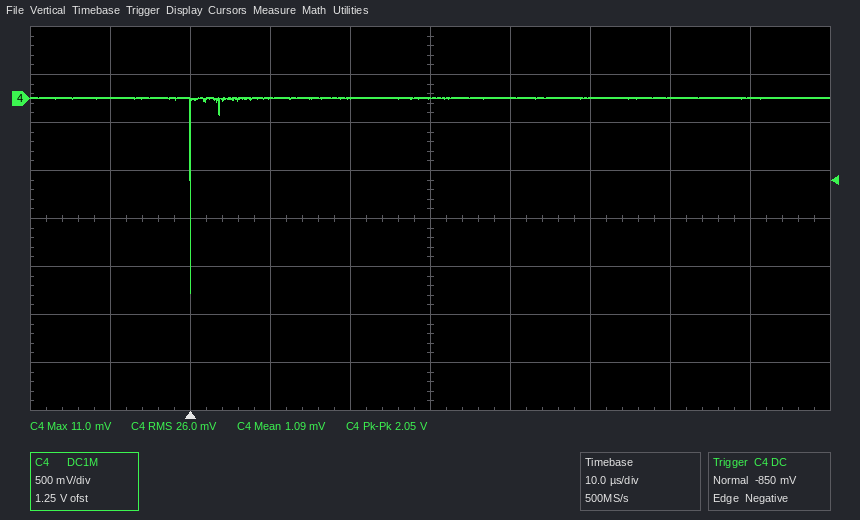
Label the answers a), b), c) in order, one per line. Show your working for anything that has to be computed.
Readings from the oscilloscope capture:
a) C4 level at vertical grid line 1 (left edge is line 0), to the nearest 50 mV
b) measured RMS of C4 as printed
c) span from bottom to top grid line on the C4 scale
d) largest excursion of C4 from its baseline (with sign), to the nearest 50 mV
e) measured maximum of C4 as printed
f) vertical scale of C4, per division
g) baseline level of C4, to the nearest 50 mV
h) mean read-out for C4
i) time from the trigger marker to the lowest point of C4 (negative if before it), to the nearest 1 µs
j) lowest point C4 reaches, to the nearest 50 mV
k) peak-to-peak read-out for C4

a) 0 mV
b) 26.0 mV
c) 4 V
d) -2.05 V − (0 mV) = -2.05 V
e) 11.0 mV
f) 500 mV
g) 0 mV
h) 1.09 mV
i) 0 µs
j) -2.05 V
k) 2.05 V
